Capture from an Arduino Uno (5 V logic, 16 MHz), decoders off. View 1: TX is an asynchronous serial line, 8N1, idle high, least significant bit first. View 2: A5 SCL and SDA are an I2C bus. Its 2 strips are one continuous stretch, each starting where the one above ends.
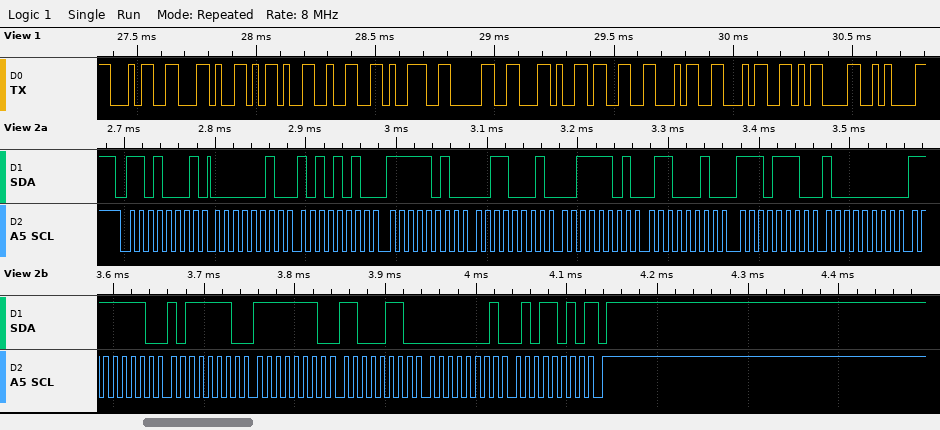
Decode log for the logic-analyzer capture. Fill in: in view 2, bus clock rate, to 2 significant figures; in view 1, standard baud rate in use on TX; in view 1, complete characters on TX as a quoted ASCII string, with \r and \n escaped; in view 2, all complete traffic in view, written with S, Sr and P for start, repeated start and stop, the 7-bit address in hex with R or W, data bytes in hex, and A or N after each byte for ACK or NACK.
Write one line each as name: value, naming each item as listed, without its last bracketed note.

in view 2, bus clock rate, to 2 significant figures: 100 kHz
in view 1, standard baud rate in use on TX: 38400 baud
in view 1, complete characters on TX as a quoted ASCII string, with \r and \n escaped: "4,-290,344\r\n"
in view 2, all complete traffic in view, written with S, Sr and P for start, repeated start and stop, the 7-bit address in hex with R or W, data bytes in hex, and A or N after each byte for ACK or NACK: S 68R A 02 A AA A FA A 31 A 3D A 62 A EE A 80 A FE A BE A FE A C6 A 01 A 5A N P
